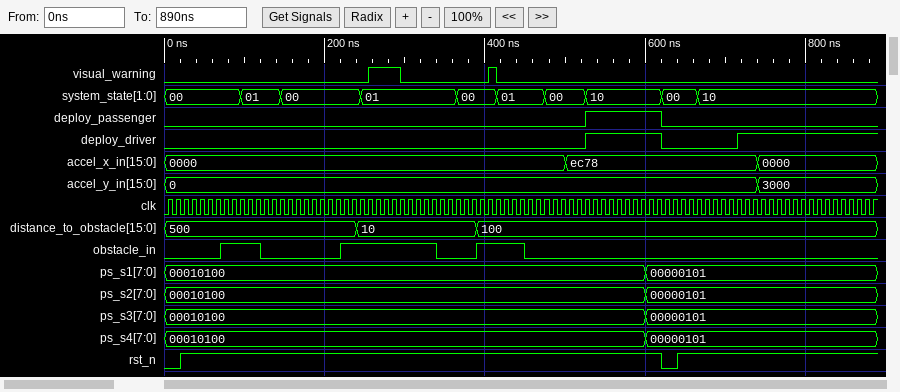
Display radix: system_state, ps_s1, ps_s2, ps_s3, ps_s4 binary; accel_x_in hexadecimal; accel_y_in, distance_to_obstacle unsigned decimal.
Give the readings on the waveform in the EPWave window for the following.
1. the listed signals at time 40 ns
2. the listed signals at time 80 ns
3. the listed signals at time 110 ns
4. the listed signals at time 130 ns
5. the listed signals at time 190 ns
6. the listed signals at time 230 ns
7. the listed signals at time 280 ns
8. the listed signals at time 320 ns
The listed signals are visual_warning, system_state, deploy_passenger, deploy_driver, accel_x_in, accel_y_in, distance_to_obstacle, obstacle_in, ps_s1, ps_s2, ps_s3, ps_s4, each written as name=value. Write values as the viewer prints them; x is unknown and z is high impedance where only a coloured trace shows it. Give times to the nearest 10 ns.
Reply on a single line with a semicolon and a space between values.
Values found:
visual_warning=0, system_state=00, deploy_passenger=0, deploy_driver=0, accel_x_in=0000, accel_y_in=0, distance_to_obstacle=500, obstacle_in=0, ps_s1=00010100, ps_s2=00010100, ps_s3=00010100, ps_s4=00010100; visual_warning=0, system_state=00, deploy_passenger=0, deploy_driver=0, accel_x_in=0000, accel_y_in=0, distance_to_obstacle=500, obstacle_in=1, ps_s1=00010100, ps_s2=00010100, ps_s3=00010100, ps_s4=00010100; visual_warning=0, system_state=01, deploy_passenger=0, deploy_driver=0, accel_x_in=0000, accel_y_in=0, distance_to_obstacle=500, obstacle_in=1, ps_s1=00010100, ps_s2=00010100, ps_s3=00010100, ps_s4=00010100; visual_warning=0, system_state=01, deploy_passenger=0, deploy_driver=0, accel_x_in=0000, accel_y_in=0, distance_to_obstacle=500, obstacle_in=0, ps_s1=00010100, ps_s2=00010100, ps_s3=00010100, ps_s4=00010100; visual_warning=0, system_state=00, deploy_passenger=0, deploy_driver=0, accel_x_in=0000, accel_y_in=0, distance_to_obstacle=500, obstacle_in=0, ps_s1=00010100, ps_s2=00010100, ps_s3=00010100, ps_s4=00010100; visual_warning=0, system_state=00, deploy_passenger=0, deploy_driver=0, accel_x_in=0000, accel_y_in=0, distance_to_obstacle=500, obstacle_in=1, ps_s1=00010100, ps_s2=00010100, ps_s3=00010100, ps_s4=00010100; visual_warning=1, system_state=01, deploy_passenger=0, deploy_driver=0, accel_x_in=0000, accel_y_in=0, distance_to_obstacle=10, obstacle_in=1, ps_s1=00010100, ps_s2=00010100, ps_s3=00010100, ps_s4=00010100; visual_warning=0, system_state=01, deploy_passenger=0, deploy_driver=0, accel_x_in=0000, accel_y_in=0, distance_to_obstacle=10, obstacle_in=1, ps_s1=00010100, ps_s2=00010100, ps_s3=00010100, ps_s4=00010100
